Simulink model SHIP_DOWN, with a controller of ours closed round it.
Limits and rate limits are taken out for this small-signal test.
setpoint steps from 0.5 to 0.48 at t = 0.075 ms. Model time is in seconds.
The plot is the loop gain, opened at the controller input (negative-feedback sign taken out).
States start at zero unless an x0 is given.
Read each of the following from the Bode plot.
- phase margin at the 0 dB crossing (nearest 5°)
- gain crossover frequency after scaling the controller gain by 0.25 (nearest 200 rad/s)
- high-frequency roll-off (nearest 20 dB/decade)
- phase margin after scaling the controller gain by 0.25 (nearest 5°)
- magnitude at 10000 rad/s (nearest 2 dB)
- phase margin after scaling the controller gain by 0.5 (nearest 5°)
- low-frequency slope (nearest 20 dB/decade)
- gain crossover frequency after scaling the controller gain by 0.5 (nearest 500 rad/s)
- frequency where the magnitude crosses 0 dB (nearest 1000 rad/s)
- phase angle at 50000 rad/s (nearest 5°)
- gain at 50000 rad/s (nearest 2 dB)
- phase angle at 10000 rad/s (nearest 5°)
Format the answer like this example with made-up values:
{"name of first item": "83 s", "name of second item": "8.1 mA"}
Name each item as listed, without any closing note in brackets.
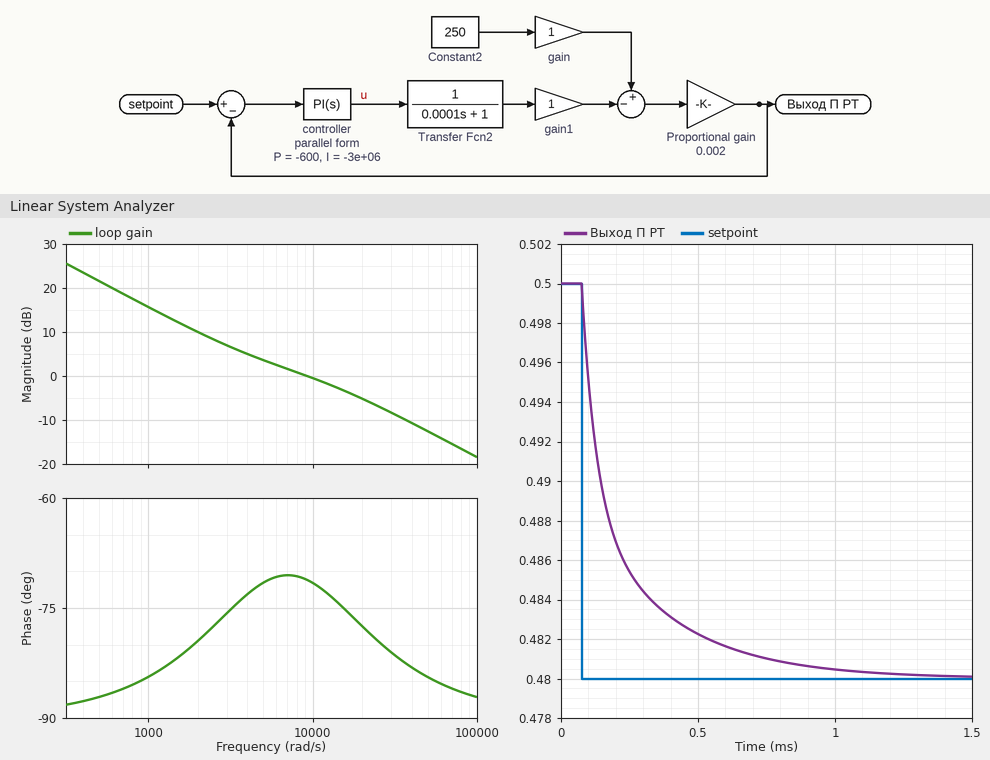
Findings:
{"phase margin at the 0 dB crossing": "110°", "gain crossover frequency after scaling the controller gain by 0.25": "1600 rad/s", "high-frequency roll-off": "-20 dB/decade", "phase margin after scaling the controller gain by 0.25": "100°", "magnitude at 10000 rad/s": "0 dB", "phase margin after scaling the controller gain by 0.5": "105°", "low-frequency slope": "-20 dB/decade", "gain crossover frequency after scaling the controller gain by 0.5": "3500 rad/s", "frequency where the magnitude crosses 0 dB": "9000 rad/s", "phase angle at 50000 rad/s": "-85°", "gain at 50000 rad/s": "-12 dB", "phase angle at 10000 rad/s": "-70°"}
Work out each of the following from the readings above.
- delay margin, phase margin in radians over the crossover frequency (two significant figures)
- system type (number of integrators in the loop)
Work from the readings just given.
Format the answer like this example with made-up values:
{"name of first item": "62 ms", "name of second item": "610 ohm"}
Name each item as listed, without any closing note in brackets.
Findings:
{"delay margin, phase margin in radians over the crossover frequency": "0.00021 s", "system type": "1"}
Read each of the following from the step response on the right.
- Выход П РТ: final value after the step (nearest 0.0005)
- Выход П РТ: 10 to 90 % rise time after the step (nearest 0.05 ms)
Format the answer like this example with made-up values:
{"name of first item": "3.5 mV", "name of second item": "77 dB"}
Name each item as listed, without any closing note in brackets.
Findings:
{"Выход П РТ: final value after the step": "0.4800", "Выход П РТ: 10 to 90 % rise time after the step": "0.45 ms"}
